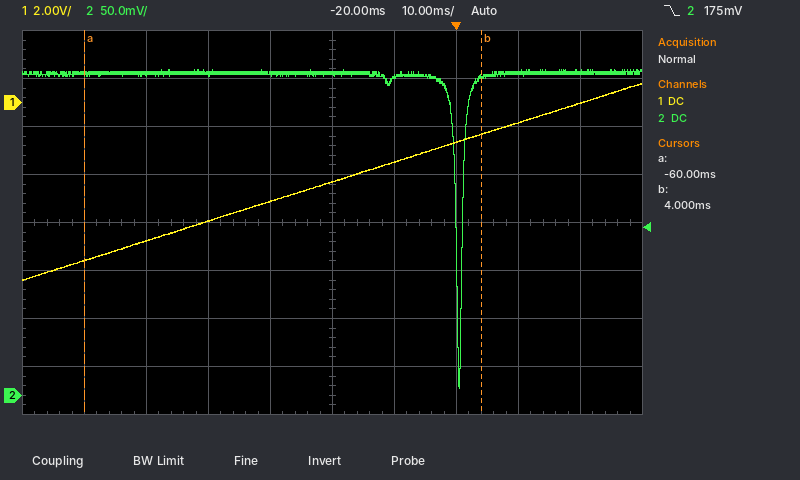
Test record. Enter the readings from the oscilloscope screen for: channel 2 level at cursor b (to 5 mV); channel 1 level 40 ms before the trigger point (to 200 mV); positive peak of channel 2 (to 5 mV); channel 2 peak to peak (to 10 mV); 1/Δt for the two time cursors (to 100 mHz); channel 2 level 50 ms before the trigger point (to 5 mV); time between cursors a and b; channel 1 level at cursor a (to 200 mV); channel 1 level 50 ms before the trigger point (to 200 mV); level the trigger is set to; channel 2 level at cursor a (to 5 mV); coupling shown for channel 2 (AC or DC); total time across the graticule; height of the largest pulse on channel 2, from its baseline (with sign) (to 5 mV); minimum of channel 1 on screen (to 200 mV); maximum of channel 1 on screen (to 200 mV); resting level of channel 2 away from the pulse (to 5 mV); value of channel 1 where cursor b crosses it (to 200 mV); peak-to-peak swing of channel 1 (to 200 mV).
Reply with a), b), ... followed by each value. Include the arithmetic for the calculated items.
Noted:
a) 330 mV
b) -5.0 V
c) 340 mV
d) 330 mV
e) 1 / 64 ms ≈ 15.6 Hz
f) 335 mV
g) 4 ms − (-60 ms) = 64 ms
h) -6.6 V
i) -5.8 V
j) 175 mV
k) 335 mV
l) DC
m) 100 ms
n) -330 mV
o) -7.4 V
p) 800 mV
q) 335 mV
r) -1.4 V
s) 800 mV − (-7.4 V) = 8.2 V
